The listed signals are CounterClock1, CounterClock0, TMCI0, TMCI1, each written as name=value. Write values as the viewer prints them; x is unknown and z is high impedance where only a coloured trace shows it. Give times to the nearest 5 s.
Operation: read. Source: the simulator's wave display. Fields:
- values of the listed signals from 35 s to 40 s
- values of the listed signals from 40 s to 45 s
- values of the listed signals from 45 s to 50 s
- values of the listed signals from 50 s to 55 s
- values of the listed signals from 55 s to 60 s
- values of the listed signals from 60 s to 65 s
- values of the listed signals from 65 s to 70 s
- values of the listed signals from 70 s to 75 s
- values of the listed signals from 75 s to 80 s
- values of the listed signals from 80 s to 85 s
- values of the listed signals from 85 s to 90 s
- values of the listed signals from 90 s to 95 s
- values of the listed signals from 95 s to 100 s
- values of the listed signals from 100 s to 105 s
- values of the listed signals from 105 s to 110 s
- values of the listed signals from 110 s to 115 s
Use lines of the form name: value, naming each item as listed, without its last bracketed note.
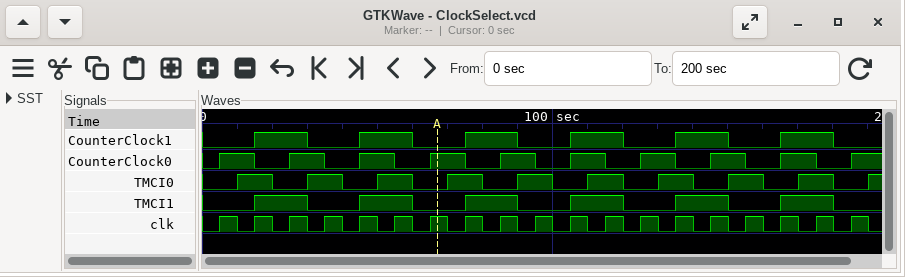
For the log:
values of the listed signals from 35 s to 40 s: CounterClock1=0, CounterClock0=0, TMCI0=1, TMCI1=0
values of the listed signals from 40 s to 45 s: CounterClock1=0, CounterClock0=0, TMCI0=0, TMCI1=0
values of the listed signals from 45 s to 50 s: CounterClock1=1, CounterClock0=1, TMCI0=0, TMCI1=1
values of the listed signals from 50 s to 55 s: CounterClock1=1, CounterClock0=1, TMCI0=1, TMCI1=1
values of the listed signals from 55 s to 60 s: CounterClock1=1, CounterClock0=0, TMCI0=1, TMCI1=1
values of the listed signals from 60 s to 65 s: CounterClock1=0, CounterClock0=0, TMCI0=0, TMCI1=0
values of the listed signals from 65 s to 70 s: CounterClock1=0, CounterClock0=1, TMCI0=0, TMCI1=0
values of the listed signals from 70 s to 75 s: CounterClock1=0, CounterClock0=1, TMCI0=1, TMCI1=0
values of the listed signals from 75 s to 80 s: CounterClock1=1, CounterClock0=0, TMCI0=1, TMCI1=1
values of the listed signals from 80 s to 85 s: CounterClock1=1, CounterClock0=0, TMCI0=0, TMCI1=1
values of the listed signals from 85 s to 90 s: CounterClock1=1, CounterClock0=1, TMCI0=0, TMCI1=1
values of the listed signals from 90 s to 95 s: CounterClock1=0, CounterClock0=1, TMCI0=1, TMCI1=0
values of the listed signals from 95 s to 100 s: CounterClock1=0, CounterClock0=0, TMCI0=1, TMCI1=0
values of the listed signals from 100 s to 105 s: CounterClock1=0, CounterClock0=0, TMCI0=0, TMCI1=0
values of the listed signals from 105 s to 110 s: CounterClock1=1, CounterClock0=1, TMCI0=0, TMCI1=1
values of the listed signals from 110 s to 115 s: CounterClock1=1, CounterClock0=1, TMCI0=1, TMCI1=1
